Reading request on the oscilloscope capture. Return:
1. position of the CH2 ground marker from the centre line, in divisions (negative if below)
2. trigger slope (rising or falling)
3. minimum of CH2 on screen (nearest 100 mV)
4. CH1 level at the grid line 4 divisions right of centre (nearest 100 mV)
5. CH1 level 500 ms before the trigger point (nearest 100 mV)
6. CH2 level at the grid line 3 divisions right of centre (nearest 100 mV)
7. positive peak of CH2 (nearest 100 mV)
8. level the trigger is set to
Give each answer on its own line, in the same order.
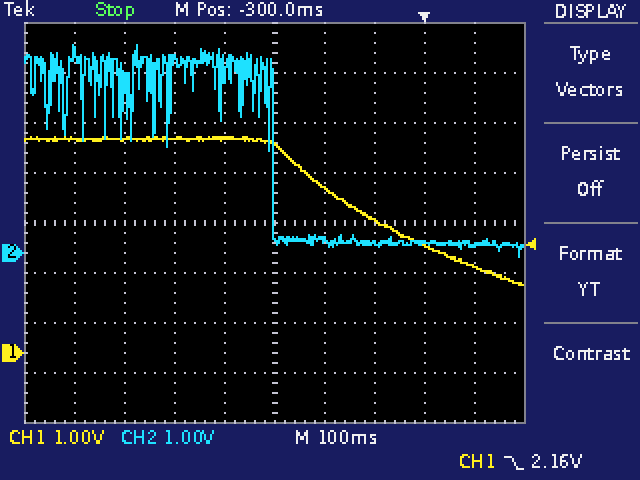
-0.6 div
falling
-100 mV
1.7 V
4.3 V
200 mV
4.2 V
2.16 V
